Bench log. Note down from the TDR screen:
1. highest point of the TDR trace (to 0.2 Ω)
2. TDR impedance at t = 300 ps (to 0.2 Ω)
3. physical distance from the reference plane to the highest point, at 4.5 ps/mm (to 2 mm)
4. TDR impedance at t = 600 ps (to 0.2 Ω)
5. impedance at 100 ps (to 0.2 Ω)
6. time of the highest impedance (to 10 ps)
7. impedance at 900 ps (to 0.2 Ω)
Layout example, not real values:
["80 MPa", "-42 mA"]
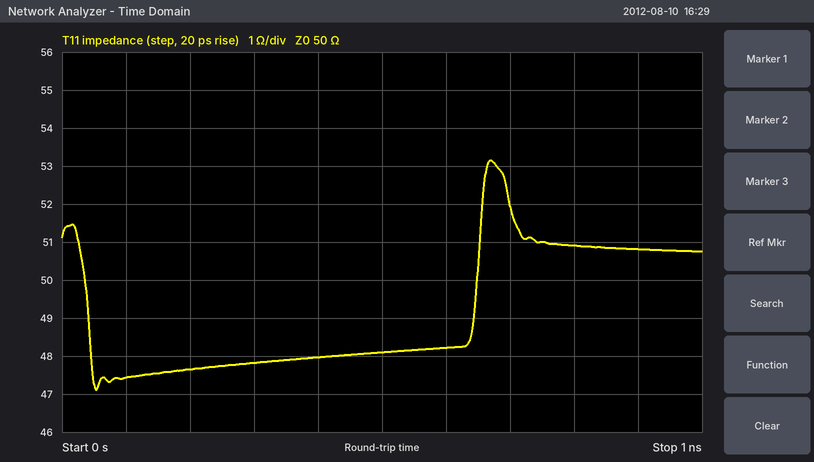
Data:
["53.2 Ω", "47.8 Ω", "74 mm", "48.2 Ω", "47.4 Ω", "670 ps", "50.8 Ω"]
